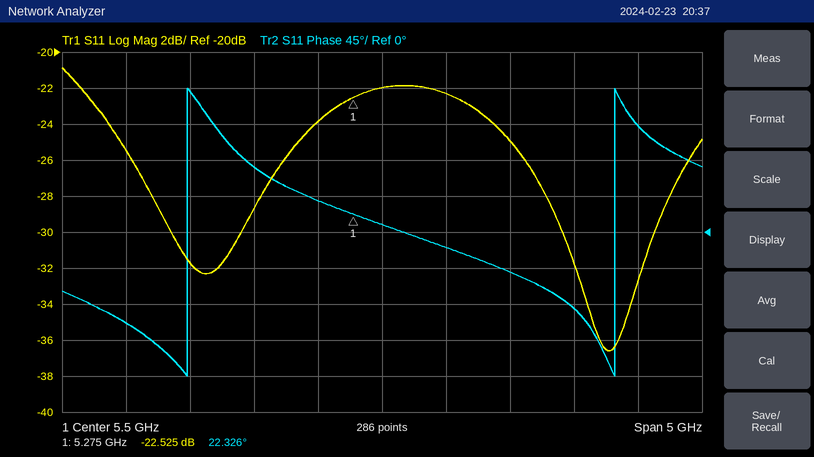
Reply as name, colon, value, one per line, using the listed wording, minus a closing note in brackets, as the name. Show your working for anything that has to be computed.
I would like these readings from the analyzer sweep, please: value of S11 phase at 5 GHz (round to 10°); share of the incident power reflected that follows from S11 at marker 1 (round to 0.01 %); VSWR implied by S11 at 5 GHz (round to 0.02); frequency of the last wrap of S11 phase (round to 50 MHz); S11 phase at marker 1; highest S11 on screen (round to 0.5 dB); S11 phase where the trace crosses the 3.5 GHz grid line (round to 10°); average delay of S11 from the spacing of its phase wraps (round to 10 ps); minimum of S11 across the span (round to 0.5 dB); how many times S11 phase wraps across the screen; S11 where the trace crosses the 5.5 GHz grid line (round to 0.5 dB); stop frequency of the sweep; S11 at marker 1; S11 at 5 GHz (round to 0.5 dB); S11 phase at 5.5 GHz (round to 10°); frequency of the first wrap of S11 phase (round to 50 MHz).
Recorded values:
value of S11 phase at 5 GHz: 40°
share of the incident power reflected that follows from S11 at marker 1: 10^(-22.525/10) ≈ 0.56 %
VSWR implied by S11 at 5 GHz: |Γ| = 10^(-24/20) = 0.0631; VSWR = (1 + 0.0631)/(1 − 0.0631) ≈ 1.13, so 1.14 to the nearest 0.02
frequency of the last wrap of S11 phase: 7.30 GHz
S11 phase at marker 1: 22.326°
highest S11 on screen: -21.0 dB
S11 phase where the trace crosses the 3.5 GHz grid line: -110°
average delay of S11 from the spacing of its phase wraps: 1 cycle / (7.30 GHz − 4.00 GHz) ≈ 303 ps, so 300 ps to the nearest 10 ps
minimum of S11 across the span: -36.5 dB
how many times S11 phase wraps across the screen: 2
S11 where the trace crosses the 5.5 GHz grid line: -22.0 dB
stop frequency of the sweep: 8 GHz
S11 at marker 1: -22.525 dB
S11 at 5 GHz: -24.0 dB
S11 phase at 5.5 GHz: 10°
frequency of the first wrap of S11 phase: 4.00 GHz
